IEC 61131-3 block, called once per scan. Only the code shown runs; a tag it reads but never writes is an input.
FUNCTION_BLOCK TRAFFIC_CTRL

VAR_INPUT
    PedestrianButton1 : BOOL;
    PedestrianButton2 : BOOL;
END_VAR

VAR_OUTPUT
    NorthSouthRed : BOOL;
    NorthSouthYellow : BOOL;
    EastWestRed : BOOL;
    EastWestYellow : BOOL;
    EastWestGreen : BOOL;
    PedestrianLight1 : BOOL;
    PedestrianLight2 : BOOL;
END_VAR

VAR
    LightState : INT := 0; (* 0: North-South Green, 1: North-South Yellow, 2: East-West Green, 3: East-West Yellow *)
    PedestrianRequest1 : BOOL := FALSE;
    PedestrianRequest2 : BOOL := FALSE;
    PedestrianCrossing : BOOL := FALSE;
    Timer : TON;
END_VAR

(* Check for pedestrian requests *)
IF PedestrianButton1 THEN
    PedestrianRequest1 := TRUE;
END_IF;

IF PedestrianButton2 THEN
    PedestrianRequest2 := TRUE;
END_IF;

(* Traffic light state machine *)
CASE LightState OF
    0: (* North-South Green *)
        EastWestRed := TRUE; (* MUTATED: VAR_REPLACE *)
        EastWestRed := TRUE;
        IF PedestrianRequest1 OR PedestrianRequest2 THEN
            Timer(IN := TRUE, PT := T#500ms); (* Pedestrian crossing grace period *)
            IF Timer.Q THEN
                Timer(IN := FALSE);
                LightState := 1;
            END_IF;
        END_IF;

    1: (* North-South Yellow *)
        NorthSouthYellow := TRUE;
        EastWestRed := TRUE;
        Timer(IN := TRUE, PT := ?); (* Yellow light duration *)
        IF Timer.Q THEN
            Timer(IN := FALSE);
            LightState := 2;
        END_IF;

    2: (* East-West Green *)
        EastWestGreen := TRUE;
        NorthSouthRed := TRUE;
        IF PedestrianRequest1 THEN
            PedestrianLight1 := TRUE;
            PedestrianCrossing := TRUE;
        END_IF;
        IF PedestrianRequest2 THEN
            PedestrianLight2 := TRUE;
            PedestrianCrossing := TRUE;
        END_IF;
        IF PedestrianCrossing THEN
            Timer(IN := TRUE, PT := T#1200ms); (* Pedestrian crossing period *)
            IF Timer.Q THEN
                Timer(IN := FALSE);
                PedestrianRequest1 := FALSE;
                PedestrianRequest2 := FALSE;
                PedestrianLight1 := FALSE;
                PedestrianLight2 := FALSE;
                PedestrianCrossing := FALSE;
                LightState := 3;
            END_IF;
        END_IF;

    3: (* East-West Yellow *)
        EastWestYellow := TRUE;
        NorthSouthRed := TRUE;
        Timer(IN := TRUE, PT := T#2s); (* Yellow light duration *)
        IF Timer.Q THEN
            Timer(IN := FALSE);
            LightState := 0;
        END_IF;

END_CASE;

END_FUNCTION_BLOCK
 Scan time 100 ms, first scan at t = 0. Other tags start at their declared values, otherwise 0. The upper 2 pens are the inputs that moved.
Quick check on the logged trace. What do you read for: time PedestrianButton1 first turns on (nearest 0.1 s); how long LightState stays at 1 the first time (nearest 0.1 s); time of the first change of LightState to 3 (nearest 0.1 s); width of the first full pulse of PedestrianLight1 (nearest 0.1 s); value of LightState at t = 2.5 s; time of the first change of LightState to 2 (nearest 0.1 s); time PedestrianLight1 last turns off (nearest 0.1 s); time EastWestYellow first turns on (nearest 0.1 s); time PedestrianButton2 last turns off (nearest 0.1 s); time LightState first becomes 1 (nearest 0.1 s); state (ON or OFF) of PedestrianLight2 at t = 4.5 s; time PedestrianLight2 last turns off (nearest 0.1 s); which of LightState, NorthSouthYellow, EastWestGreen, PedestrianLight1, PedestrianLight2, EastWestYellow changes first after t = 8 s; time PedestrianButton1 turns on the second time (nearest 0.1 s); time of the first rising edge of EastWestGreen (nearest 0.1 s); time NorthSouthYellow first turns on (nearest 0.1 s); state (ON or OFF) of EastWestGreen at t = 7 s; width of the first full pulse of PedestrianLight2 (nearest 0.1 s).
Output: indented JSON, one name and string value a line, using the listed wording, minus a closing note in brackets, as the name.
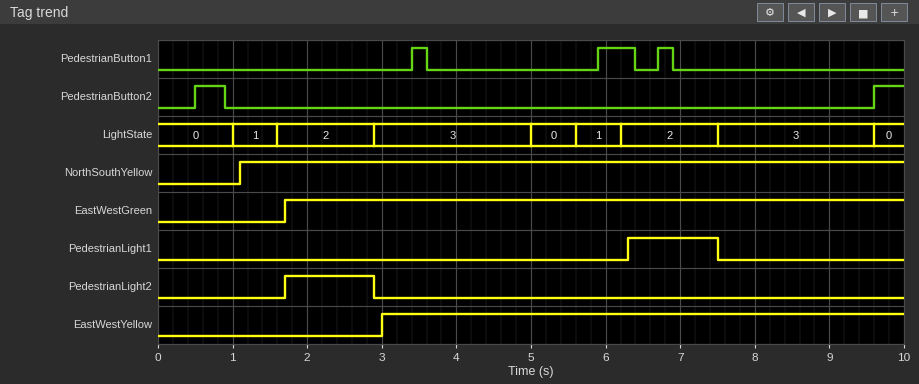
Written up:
{
  "time PedestrianButton1 first turns on": "3.4 s",
  "how long LightState stays at 1 the first time": "0.6 s",
  "time of the first change of LightState to 3": "2.9 s",
  "width of the first full pulse of PedestrianLight1": "1.2 s",
  "value of LightState at t = 2.5 s": "2",
  "time of the first change of LightState to 2": "1.6 s",
  "time PedestrianLight1 last turns off": "7.5 s",
  "time EastWestYellow first turns on": "3.0 s",
  "time PedestrianButton2 last turns off": "0.9 s",
  "time LightState first becomes 1": "1.0 s",
  "state (ON or OFF) of PedestrianLight2 at t = 4.5 s": "OFF",
  "time PedestrianLight2 last turns off": "2.9 s",
  "which of LightState, NorthSouthYellow, EastWestGreen, PedestrianLight1, PedestrianLight2, EastWestYellow changes first after t = 8 s": "LightState",
  "time PedestrianButton1 turns on the second time": "5.9 s",
  "time of the first rising edge of EastWestGreen": "1.7 s",
  "time NorthSouthYellow first turns on": "1.1 s",
  "state (ON or OFF) of EastWestGreen at t = 7 s": "ON",
  "width of the first full pulse of PedestrianLight2": "1.2 s"
}
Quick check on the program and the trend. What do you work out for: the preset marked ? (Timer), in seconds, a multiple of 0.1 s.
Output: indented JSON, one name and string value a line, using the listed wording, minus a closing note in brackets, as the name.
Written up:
{
  "the preset marked ? (Timer), in seconds, a multiple of 0.1 s": "0.5 s"
}
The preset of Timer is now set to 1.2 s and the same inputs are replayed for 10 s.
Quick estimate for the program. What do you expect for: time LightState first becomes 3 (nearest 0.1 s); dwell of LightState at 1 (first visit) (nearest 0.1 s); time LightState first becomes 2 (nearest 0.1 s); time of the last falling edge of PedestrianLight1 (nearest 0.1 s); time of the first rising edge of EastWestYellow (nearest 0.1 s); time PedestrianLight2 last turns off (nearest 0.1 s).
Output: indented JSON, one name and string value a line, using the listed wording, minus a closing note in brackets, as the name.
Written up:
{
  "time LightState first becomes 3": "3.6 s",
  "dwell of LightState at 1 (first visit)": "1.3 s",
  "time LightState first becomes 2": "2.3 s",
  "time of the last falling edge of PedestrianLight1": "9.0 s",
  "time of the first rising edge of EastWestYellow": "3.7 s",
  "time PedestrianLight2 last turns off": "3.6 s"
}
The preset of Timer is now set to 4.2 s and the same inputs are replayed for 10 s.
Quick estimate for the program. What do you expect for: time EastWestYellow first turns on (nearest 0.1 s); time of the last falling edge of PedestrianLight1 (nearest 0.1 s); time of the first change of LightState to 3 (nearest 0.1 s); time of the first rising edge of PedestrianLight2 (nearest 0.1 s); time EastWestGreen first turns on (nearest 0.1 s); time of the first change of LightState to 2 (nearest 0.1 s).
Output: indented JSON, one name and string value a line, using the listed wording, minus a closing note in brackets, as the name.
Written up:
{
  "time EastWestYellow first turns on": "6.7 s",
  "time of the last falling edge of PedestrianLight1": "6.6 s",
  "time of the first change of LightState to 3": "6.6 s",
  "time of the first rising edge of PedestrianLight2": "5.4 s",
  "time EastWestGreen first turns on": "5.4 s",
  "time of the first change of LightState to 2": "5.3 s"
}
